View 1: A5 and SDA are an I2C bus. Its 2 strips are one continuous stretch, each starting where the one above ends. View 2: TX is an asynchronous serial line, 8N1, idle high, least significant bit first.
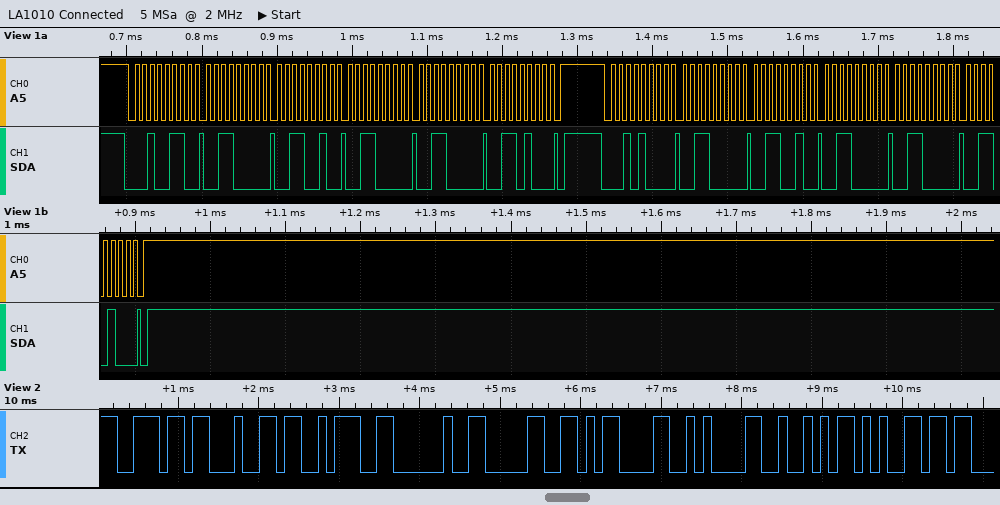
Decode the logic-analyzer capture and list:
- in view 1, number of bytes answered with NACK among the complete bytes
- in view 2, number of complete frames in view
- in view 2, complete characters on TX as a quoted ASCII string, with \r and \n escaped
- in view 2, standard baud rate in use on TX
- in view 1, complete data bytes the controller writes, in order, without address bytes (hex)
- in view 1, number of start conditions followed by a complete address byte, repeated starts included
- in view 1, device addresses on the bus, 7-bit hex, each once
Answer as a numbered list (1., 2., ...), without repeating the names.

1. 0
2. 9
3. "nd: 0\r\nRe"
4. 9600 baud
5. 30 32 30 30 34 30 32 30 30 34
6. 2
7. 0x13 0x14
